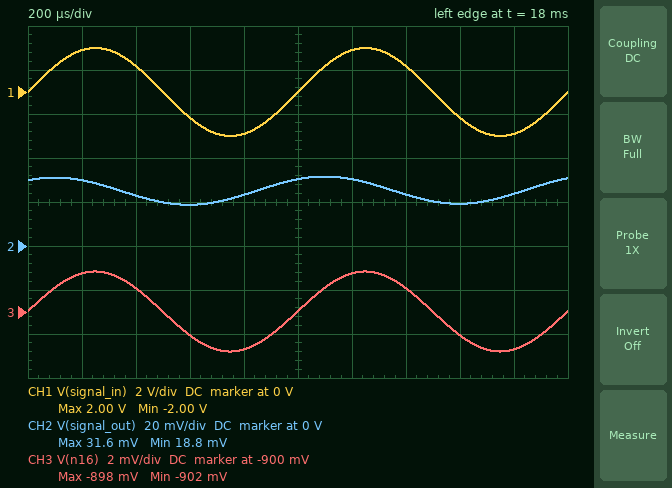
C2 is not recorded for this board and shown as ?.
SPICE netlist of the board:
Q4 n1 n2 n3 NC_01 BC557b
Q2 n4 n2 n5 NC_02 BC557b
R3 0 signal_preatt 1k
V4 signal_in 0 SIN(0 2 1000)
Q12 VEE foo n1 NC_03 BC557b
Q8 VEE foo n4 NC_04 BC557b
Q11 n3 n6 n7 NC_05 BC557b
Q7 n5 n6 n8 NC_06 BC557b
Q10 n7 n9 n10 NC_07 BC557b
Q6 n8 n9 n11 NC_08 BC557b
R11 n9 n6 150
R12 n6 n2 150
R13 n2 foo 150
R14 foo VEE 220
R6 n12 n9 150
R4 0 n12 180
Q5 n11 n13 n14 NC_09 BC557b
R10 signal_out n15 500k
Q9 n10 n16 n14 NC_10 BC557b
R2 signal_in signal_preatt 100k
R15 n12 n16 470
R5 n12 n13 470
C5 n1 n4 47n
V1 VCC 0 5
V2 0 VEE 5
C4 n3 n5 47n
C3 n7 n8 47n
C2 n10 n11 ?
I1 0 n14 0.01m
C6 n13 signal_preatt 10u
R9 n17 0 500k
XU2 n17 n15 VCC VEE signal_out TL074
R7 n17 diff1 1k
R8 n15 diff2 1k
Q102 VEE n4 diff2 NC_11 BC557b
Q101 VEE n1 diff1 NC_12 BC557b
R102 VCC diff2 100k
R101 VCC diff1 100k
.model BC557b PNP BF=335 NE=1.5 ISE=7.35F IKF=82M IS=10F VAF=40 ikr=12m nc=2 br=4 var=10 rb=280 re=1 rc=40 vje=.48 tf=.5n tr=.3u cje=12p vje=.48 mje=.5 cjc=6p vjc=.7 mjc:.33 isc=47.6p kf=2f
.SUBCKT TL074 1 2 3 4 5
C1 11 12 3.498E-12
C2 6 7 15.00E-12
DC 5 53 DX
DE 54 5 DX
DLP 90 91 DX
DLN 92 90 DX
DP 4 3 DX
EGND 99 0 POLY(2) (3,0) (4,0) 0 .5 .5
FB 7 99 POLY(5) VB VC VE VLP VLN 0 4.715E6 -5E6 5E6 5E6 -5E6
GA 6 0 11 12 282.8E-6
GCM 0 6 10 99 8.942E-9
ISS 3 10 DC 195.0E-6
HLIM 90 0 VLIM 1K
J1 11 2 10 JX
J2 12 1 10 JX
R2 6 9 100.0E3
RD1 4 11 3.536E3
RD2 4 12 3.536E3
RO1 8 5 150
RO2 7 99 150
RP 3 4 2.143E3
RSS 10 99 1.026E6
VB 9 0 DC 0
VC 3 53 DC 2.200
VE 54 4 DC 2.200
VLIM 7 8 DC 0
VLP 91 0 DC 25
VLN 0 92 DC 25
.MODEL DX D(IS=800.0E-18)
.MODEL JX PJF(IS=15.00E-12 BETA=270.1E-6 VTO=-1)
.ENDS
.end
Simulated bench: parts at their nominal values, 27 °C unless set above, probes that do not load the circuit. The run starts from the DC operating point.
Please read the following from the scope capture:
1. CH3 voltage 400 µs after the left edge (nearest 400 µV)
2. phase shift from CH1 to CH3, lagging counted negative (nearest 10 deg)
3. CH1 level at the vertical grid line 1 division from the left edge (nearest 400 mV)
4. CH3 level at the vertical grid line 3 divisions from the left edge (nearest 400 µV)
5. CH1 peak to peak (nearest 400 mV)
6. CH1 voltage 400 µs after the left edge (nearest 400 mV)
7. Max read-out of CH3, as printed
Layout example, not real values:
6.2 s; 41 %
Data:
-898.8 mV; 0 deg; 2.0 V; -901.2 mV; 4.0 V; 1.2 V; -898 mV
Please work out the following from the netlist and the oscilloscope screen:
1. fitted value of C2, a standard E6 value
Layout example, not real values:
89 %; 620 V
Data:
150 nF
